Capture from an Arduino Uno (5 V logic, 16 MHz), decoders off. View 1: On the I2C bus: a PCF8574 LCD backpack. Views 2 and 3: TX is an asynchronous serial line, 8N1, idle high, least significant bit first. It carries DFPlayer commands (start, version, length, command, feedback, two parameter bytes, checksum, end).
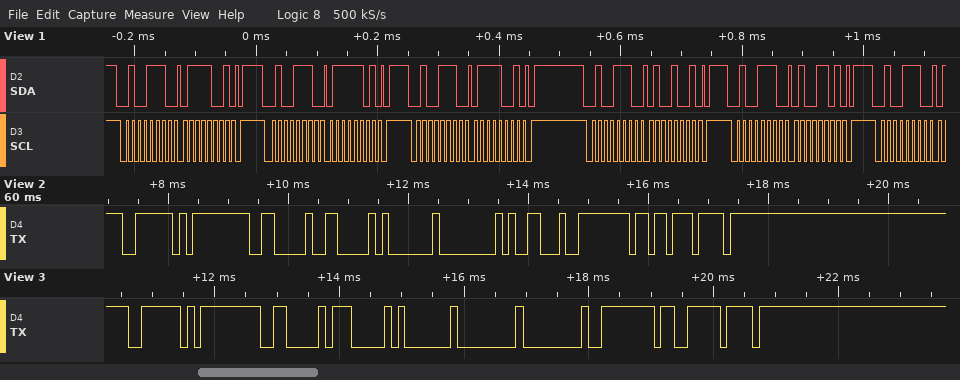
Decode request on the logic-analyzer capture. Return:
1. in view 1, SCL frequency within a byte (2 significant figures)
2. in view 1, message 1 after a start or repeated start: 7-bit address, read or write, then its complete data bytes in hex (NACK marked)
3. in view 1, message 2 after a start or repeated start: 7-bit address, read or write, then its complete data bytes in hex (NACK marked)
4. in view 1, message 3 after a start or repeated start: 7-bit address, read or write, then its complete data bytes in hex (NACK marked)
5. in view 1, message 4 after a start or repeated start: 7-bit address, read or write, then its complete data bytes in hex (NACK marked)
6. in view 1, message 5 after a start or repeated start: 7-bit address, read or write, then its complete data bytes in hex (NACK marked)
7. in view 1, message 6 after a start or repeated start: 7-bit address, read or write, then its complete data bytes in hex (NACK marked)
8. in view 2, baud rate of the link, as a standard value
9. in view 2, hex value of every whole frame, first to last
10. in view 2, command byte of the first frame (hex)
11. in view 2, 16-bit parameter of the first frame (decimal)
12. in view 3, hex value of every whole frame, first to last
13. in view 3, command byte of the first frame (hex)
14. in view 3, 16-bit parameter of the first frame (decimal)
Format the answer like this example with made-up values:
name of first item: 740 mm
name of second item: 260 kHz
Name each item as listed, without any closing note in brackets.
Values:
in view 1, SCL frequency within a byte: 100 kHz
in view 1, message 1 after a start or repeated start: 7-bit address, read or write, then its complete data bytes in hex: 0x27 write: 79
in view 1, message 2 after a start or repeated start: 7-bit address, read or write, then its complete data bytes in hex: 0x27 write: 7D
in view 1, message 3 after a start or repeated start: 7-bit address, read or write, then its complete data bytes in hex: 0x27 write: 79
in view 1, message 4 after a start or repeated start: 7-bit address, read or write, then its complete data bytes in hex: 0x27 write: 49
in view 1, message 5 after a start or repeated start: 7-bit address, read or write, then its complete data bytes in hex: 0x27 write: 4D
in view 1, message 6 after a start or repeated start: 7-bit address, read or write, then its complete data bytes in hex: 0x27 write
in view 2, baud rate of the link, as a standard value: 9600 baud
in view 2, hex value of every whole frame, first to last: 7E FF 06 06 01 00 19 FE DB EF
in view 2, command byte of the first frame: 0x06
in view 2, 16-bit parameter of the first frame: 25
in view 3, hex value of every whole frame, first to last: 0x7E 0xFF 0x06 0x07 0x01 0x00 0x00 0xFE 0xF3 0xEF
in view 3, command byte of the first frame: 0x07
in view 3, 16-bit parameter of the first frame: 0
